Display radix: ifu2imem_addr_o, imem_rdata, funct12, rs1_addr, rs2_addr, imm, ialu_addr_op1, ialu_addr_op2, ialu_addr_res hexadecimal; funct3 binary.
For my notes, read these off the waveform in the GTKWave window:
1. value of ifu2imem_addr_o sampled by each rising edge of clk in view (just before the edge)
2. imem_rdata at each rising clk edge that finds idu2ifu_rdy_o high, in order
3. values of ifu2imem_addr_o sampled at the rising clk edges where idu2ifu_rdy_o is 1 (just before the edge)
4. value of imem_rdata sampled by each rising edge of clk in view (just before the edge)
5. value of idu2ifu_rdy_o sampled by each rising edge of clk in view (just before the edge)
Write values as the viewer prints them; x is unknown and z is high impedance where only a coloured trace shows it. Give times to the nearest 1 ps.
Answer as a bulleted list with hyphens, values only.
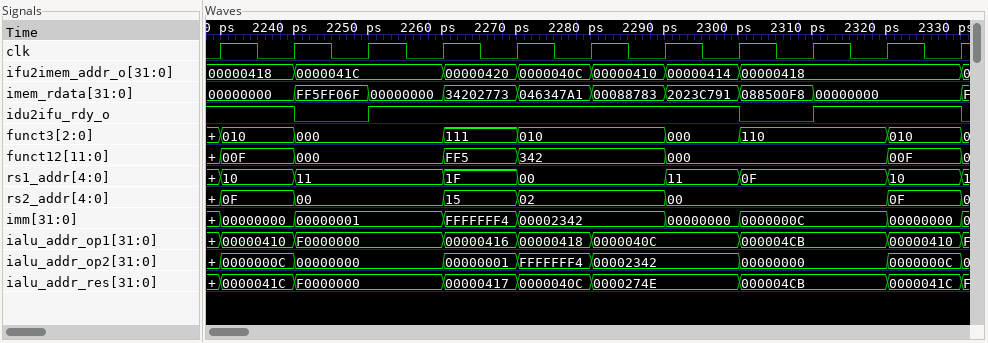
- 00000418, 00000418, 0000041C, 0000041C, 00000420, 0000040C, 00000410, 00000414, 00000418, 00000418, 00000418
- 00000000, 00000000, 00000000, 34202773, 046347A1, 00088783, 2023C791, 00000000, 00000000
- 00000418, 00000418, 0000041C, 00000420, 0000040C, 00000410, 00000414, 00000418, 00000418
- 00000000, 00000000, FF5FF06F, 00000000, 34202773, 046347A1, 00088783, 2023C791, 088500F8, 00000000, 00000000
- 1 1 0 1 1 1 1 1 0 1 1
